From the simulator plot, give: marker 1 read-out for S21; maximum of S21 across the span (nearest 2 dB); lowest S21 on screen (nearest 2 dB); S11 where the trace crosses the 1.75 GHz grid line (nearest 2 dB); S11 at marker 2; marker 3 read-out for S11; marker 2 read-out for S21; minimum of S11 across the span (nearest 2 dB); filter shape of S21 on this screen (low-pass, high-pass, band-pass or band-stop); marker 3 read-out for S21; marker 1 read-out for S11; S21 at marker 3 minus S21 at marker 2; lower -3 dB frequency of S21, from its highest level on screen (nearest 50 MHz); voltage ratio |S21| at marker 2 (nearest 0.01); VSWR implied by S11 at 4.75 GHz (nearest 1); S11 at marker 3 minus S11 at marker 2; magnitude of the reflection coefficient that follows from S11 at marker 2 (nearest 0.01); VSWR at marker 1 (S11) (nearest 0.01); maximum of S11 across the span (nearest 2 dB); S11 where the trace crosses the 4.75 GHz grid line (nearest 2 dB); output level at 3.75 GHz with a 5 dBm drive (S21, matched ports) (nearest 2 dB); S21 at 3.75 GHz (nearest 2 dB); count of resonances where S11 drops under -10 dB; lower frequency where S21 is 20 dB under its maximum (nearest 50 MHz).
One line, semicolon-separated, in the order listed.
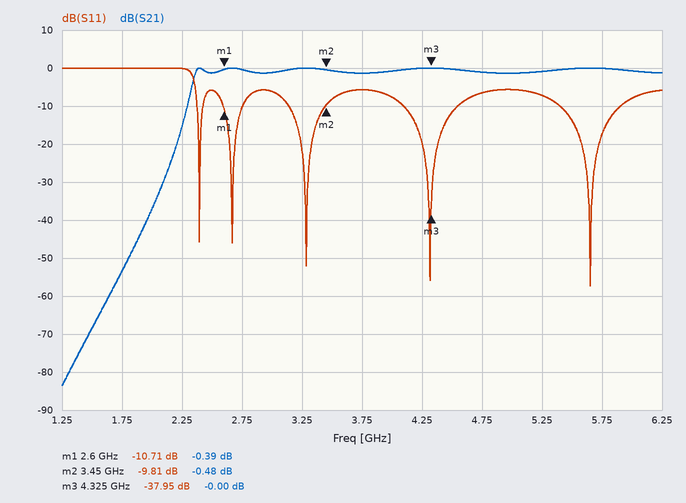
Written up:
-0.39 dB; 0 dB; -84 dB; 0 dB; -9.81 dB; -37.95 dB; -0.48 dB; -58 dB; high-pass; -0.00 dB; -10.71 dB; 0.48 dB; 2.35 GHz; 0.95; 3; -28.14 dB; 0.32; 1.82; 0 dB; -6 dB; 4 dBm; -2 dB; 5; 2.20 GHz
